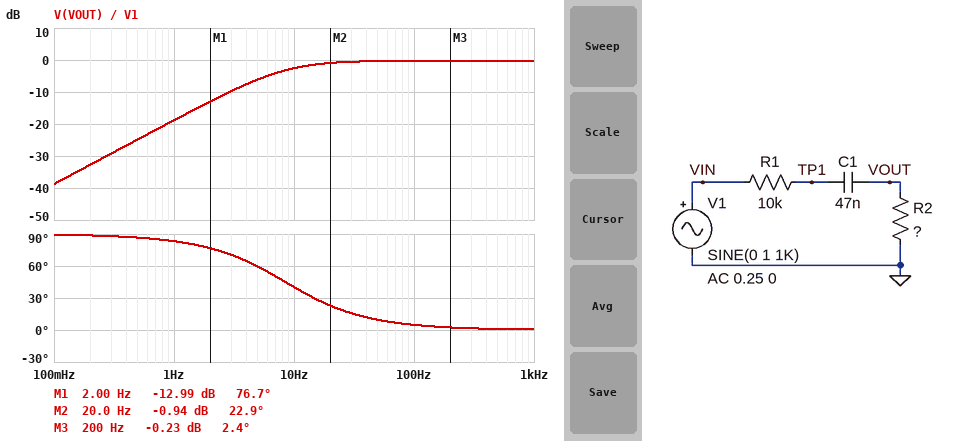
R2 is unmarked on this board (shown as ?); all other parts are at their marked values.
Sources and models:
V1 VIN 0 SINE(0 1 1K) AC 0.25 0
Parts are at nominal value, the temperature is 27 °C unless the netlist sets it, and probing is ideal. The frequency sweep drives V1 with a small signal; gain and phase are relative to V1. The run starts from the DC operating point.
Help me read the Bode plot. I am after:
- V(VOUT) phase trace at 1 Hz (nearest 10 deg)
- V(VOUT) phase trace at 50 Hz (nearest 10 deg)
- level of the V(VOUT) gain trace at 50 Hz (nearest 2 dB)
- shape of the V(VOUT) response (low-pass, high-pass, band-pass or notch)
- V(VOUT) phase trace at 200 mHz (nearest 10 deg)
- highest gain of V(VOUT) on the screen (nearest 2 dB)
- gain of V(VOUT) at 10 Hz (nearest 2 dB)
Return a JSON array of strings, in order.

["80 deg", "10 deg", "0 dB", "high-pass", "90 deg", "0 dB", "-2 dB"]
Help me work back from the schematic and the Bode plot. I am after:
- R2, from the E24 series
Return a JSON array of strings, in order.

["390 kΩ"]
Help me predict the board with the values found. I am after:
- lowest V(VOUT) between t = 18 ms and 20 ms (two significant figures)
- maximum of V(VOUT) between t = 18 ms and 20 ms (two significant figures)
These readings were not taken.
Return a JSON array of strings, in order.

["-980 mV", "970 mV"]
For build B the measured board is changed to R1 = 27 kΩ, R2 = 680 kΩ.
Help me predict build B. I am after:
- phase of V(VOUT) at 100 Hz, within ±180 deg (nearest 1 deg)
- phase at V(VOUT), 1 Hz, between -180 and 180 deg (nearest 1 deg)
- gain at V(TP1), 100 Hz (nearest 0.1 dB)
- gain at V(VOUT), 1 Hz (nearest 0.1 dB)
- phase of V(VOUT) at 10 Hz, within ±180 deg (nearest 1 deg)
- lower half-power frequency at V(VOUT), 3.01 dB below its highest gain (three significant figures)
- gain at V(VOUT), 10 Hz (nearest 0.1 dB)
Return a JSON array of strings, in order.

["3 deg", "78 deg", "-0.3 dB", "-14.1 dB", "26 deg", "4.79 Hz", "-1.2 dB"]
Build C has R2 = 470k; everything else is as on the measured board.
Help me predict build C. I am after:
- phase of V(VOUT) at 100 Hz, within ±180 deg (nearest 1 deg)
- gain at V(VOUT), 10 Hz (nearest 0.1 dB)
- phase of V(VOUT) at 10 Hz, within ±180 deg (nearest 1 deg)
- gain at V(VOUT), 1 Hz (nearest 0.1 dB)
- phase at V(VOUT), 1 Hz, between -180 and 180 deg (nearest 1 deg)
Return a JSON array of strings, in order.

["4 deg", "-1.9 dB", "35 deg", "-17.2 dB", "82 deg"]
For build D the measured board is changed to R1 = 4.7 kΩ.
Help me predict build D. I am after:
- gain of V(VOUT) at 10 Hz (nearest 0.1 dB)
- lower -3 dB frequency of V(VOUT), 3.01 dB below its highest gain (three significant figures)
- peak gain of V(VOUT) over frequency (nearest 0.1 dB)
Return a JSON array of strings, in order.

["-2.5 dB", "8.58 Hz", "-0.1 dB"]
